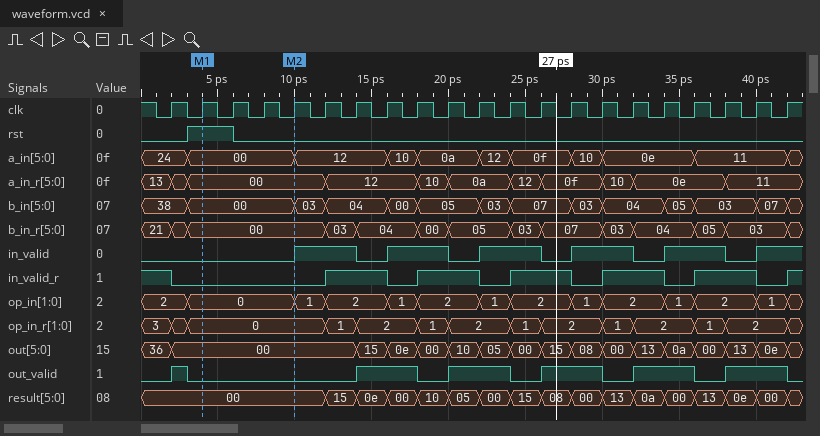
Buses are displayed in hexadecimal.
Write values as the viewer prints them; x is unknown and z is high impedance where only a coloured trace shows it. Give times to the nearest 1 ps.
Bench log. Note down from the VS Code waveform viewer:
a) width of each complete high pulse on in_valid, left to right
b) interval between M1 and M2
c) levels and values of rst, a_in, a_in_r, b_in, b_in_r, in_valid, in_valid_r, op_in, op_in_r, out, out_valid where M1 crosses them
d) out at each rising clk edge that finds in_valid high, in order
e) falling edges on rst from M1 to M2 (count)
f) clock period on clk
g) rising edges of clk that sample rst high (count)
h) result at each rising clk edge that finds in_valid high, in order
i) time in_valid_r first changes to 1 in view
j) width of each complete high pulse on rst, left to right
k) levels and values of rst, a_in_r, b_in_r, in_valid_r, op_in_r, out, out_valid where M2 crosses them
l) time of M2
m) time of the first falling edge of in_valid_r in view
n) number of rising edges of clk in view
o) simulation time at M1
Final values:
4 ps, 4 ps, 4 ps, 4 ps, 4 ps
6 ps
rst=1, a_in=00, a_in_r=00, b_in=00, b_in_r=00, in_valid=0, in_valid_r=0, op_in=0, op_in_r=0, out=00, out_valid=0
00, 00, 0e, 00, 05, 00, 08, 00, 0a, 00, 0e
1
2 ps
2
00, 15, 00, 10, 00, 15, 00, 13, 00, 13, 00
12 ps
3 ps
rst=0, a_in_r=00, b_in_r=00, in_valid_r=0, op_in_r=0, out=00, out_valid=0
10 ps
2 ps
21
4 ps
